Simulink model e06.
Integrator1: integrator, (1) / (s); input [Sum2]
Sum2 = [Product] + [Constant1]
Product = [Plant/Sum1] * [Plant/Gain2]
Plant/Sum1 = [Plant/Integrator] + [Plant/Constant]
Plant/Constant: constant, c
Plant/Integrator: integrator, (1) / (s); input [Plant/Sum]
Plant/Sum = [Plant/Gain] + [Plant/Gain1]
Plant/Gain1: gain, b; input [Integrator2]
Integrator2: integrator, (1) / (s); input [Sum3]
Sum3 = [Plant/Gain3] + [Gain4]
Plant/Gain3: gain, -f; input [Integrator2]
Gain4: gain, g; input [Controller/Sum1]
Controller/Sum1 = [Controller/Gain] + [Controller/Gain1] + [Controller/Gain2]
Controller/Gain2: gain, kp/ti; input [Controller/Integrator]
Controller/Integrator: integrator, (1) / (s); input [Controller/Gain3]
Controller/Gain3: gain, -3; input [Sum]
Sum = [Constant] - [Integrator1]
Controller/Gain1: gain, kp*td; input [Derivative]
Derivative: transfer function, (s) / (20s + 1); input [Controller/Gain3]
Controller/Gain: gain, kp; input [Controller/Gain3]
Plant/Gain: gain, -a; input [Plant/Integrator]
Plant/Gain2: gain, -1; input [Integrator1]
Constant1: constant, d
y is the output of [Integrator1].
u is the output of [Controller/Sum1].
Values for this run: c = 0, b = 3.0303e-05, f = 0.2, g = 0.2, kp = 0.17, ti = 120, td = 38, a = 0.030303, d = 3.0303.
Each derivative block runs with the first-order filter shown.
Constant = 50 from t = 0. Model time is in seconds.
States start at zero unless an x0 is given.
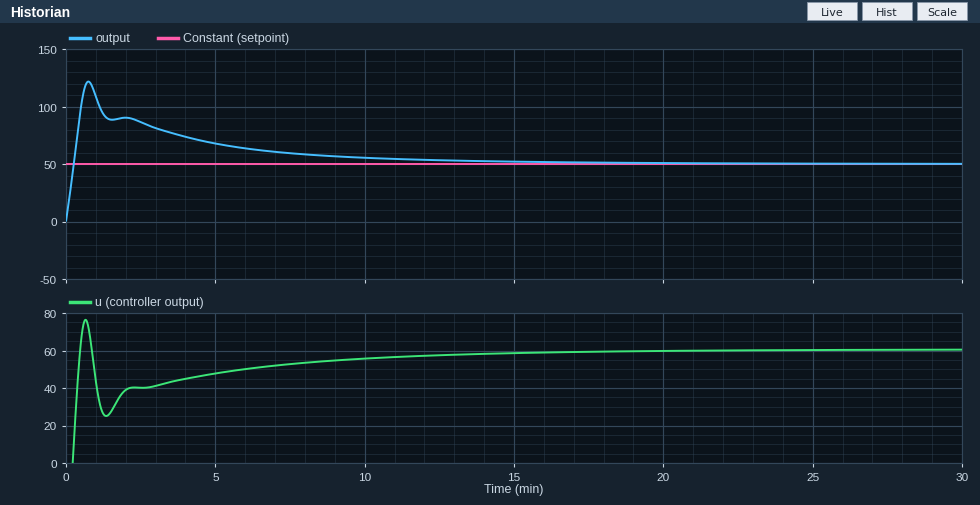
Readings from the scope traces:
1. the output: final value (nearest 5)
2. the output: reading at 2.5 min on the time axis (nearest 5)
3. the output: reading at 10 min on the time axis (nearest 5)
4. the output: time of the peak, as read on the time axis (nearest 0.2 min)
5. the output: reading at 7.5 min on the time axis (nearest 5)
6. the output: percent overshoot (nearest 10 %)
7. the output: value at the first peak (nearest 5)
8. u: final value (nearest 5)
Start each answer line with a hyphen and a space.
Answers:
- 50
- 85
- 55
- 0.8 min
- 60
- 140 %
- 120
- 60
